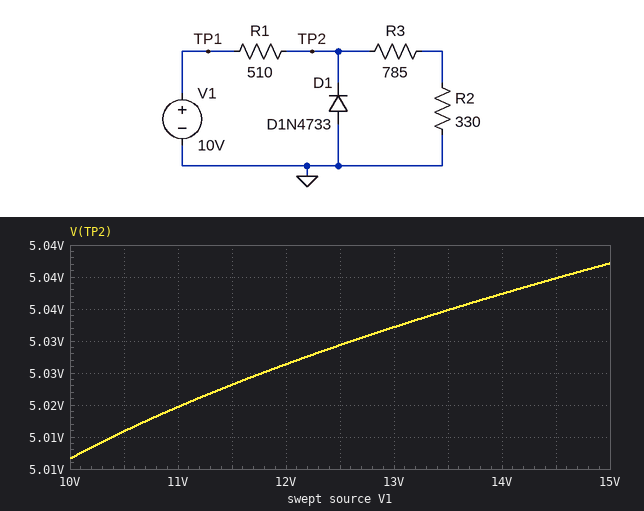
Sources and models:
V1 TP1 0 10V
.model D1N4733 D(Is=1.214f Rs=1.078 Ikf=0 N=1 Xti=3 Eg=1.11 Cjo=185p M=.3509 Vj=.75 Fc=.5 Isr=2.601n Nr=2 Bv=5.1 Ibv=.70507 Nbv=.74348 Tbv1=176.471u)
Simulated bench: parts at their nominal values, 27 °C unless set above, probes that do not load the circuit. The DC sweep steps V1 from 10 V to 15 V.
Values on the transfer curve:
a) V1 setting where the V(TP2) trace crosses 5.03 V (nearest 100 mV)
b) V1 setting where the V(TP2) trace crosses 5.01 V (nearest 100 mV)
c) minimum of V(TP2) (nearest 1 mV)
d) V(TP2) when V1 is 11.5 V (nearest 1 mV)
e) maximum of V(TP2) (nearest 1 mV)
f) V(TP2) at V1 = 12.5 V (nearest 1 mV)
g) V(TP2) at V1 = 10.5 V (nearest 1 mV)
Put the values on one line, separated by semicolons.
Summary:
11.8 V; 10.4 V; 5.012 V; 5.023 V; 5.042 V; 5.029 V; 5.016 V
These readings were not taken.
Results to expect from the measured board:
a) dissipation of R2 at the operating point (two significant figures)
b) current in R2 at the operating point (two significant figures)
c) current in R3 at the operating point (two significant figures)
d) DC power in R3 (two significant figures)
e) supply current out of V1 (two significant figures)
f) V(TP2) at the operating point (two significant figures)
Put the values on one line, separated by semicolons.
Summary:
6.7 mW; 4.5 mA; 4.5 mA; 16 mW; 9.8 mA; 5.0 V
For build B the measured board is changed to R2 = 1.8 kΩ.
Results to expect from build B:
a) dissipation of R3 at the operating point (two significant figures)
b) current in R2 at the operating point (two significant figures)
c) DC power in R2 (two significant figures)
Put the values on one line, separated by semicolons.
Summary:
3.0 mW; 1.9 mA; 6.8 mW
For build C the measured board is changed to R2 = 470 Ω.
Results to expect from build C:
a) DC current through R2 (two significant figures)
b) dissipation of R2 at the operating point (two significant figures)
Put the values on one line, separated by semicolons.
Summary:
4.0 mA; 7.5 mW
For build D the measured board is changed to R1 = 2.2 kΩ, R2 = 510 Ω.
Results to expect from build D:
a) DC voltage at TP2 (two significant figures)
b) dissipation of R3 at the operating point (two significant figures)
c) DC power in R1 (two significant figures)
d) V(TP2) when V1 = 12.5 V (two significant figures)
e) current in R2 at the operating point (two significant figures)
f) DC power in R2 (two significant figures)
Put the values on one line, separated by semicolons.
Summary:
3.7 V; 6.4 mW; 18 mW; 4.6 V; 2.9 mA; 4.2 mW
